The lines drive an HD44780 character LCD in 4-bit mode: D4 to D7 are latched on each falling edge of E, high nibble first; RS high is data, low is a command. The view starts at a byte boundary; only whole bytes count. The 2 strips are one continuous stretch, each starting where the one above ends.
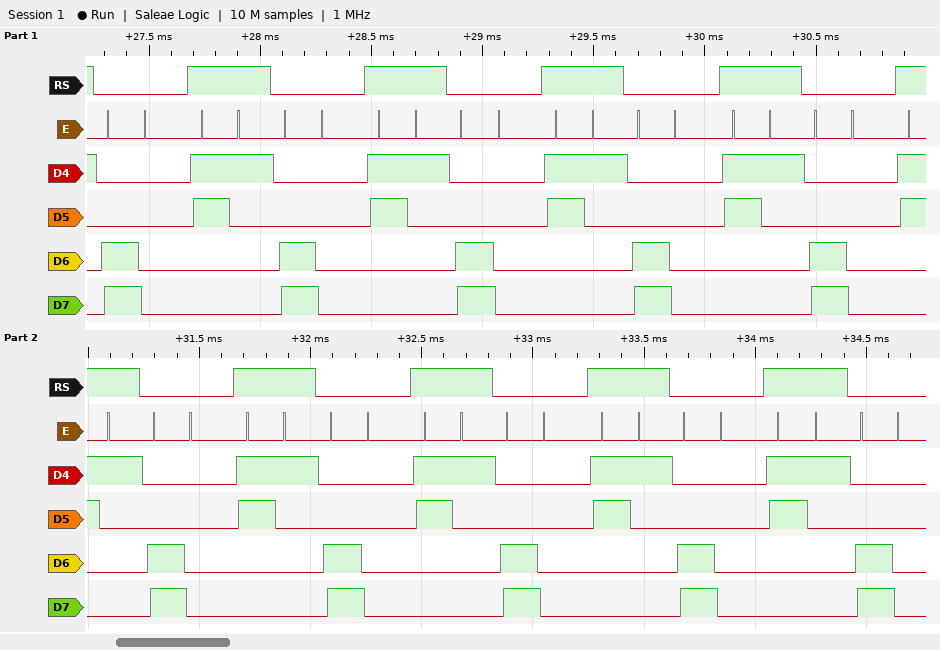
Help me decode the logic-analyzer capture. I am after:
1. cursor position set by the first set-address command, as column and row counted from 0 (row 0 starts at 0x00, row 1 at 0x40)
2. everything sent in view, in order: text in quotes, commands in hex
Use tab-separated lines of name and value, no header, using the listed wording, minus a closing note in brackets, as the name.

cursor position set by the first set-address command, as column and row counted from 0	column 0, row 1
everything sent in view, in order: text in quotes, commands in hex	0xC0 "1" 0xC0 "1" 0xC0 "1" 0xC0 "1" 0xC0 "1" 0xC0 "1" 0xC0 "1" 0xC0 "1" 0xC0 "1" 0xC0
